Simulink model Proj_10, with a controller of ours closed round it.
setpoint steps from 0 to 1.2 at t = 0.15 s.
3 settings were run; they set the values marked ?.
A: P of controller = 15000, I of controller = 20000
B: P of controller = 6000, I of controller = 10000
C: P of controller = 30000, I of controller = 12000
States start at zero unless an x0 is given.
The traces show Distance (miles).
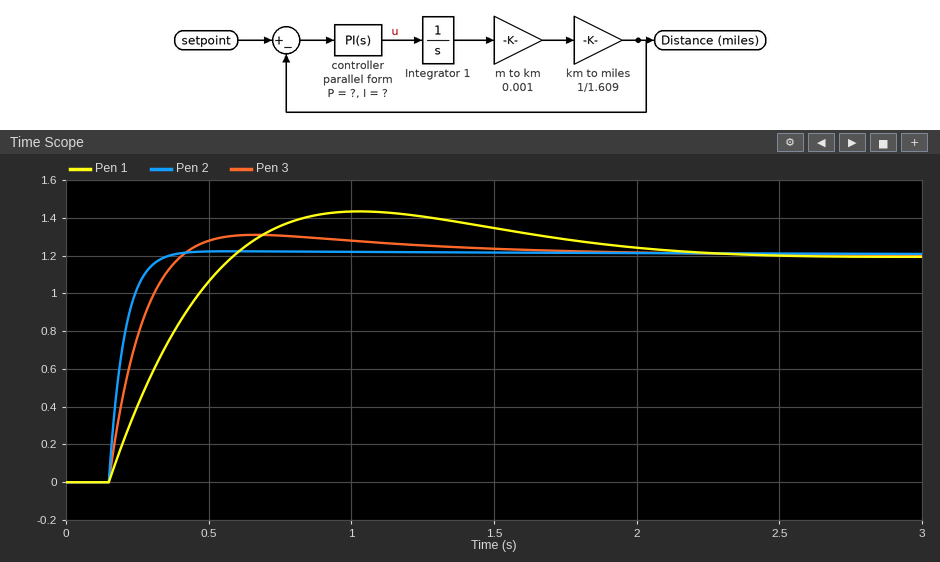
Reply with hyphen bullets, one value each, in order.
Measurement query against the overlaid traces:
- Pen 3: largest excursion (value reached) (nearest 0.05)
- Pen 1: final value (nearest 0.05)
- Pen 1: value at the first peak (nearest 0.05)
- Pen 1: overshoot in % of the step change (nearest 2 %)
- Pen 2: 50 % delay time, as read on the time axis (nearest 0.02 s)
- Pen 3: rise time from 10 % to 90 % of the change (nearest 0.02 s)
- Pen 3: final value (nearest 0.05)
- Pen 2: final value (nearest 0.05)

- 1.30
- 1.20
- 1.45
- 20 %
- 0.18 s
- 0.18 s
- 1.20
- 1.20
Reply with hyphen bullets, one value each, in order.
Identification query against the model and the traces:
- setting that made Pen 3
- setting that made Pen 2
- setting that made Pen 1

- A
- C
- B
